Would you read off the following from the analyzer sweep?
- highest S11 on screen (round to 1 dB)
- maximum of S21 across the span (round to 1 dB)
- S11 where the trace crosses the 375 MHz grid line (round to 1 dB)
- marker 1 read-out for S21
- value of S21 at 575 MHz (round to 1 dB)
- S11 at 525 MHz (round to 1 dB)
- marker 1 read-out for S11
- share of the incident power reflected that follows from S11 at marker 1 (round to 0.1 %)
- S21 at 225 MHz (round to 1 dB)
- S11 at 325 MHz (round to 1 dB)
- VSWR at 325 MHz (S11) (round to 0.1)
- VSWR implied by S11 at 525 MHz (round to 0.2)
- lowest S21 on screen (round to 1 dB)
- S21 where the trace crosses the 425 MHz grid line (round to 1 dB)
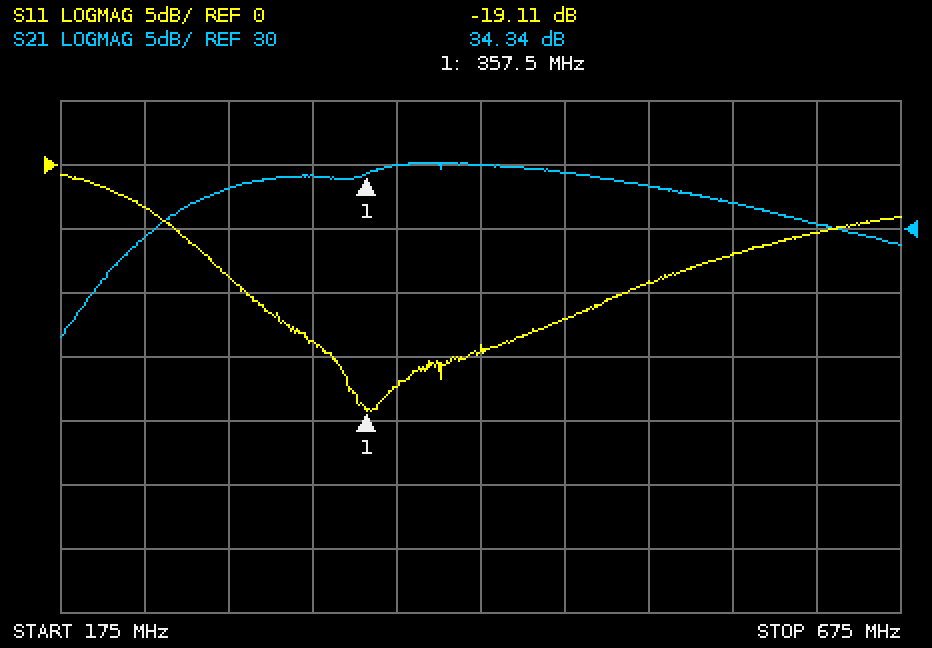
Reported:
-1 dB
35 dB
-17 dB
34.34 dB
32 dB
-9 dB
-19.11 dB
1.2 %
29 dB
-14 dB
1.5
2.0
22 dB
35 dB
